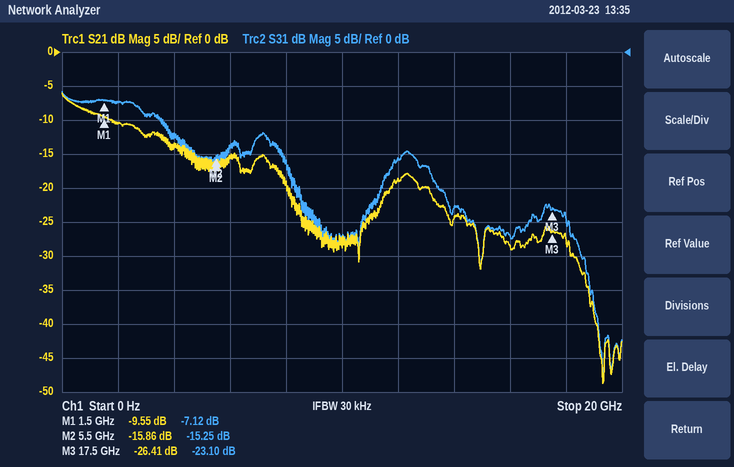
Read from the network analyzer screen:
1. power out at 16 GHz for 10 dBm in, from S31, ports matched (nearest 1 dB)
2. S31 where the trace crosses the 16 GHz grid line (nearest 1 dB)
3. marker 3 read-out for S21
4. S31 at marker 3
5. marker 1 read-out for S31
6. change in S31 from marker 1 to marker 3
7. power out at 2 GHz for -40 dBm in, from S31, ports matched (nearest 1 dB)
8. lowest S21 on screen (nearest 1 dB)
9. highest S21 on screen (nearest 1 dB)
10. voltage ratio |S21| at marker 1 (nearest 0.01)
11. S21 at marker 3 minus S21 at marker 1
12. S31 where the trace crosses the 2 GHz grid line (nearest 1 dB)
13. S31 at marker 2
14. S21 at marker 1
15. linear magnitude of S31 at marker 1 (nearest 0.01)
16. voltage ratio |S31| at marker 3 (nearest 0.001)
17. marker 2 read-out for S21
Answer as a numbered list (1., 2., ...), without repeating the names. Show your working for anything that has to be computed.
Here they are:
1. 10 dBm + (-27 dB) = -17 dBm
2. -27 dB
3. -26.41 dB
4. -23.10 dB
5. -7.12 dB
6. -23.1 − (-7.12) = -15.98 dB
7. -40 dBm + (-7 dB) = -47 dBm
8. -49 dB
9. -6 dB
10. 10^(-9.55/20) ≈ 0.33
11. -26.41 − (-9.55) = -16.86 dB
12. -7 dB
13. -15.25 dB
14. -9.55 dB
15. 10^(-7.12/20) ≈ 0.44
16. 10^(-23.1/20) ≈ 0.070
17. -15.86 dB
